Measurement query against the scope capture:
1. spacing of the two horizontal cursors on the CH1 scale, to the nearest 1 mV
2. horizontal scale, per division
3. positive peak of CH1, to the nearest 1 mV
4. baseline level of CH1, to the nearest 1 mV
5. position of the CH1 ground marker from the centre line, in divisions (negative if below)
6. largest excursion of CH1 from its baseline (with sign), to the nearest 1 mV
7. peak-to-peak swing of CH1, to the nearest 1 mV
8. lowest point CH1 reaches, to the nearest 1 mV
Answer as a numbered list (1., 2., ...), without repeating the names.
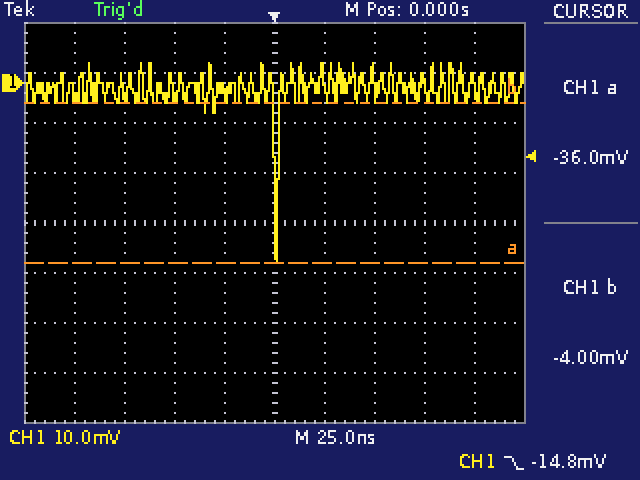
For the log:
1. 32 mV
2. 25 ns
3. 4 mV
4. -1 mV
5. +2.8 div
6. -35 mV
7. 40 mV
8. -36 mV
